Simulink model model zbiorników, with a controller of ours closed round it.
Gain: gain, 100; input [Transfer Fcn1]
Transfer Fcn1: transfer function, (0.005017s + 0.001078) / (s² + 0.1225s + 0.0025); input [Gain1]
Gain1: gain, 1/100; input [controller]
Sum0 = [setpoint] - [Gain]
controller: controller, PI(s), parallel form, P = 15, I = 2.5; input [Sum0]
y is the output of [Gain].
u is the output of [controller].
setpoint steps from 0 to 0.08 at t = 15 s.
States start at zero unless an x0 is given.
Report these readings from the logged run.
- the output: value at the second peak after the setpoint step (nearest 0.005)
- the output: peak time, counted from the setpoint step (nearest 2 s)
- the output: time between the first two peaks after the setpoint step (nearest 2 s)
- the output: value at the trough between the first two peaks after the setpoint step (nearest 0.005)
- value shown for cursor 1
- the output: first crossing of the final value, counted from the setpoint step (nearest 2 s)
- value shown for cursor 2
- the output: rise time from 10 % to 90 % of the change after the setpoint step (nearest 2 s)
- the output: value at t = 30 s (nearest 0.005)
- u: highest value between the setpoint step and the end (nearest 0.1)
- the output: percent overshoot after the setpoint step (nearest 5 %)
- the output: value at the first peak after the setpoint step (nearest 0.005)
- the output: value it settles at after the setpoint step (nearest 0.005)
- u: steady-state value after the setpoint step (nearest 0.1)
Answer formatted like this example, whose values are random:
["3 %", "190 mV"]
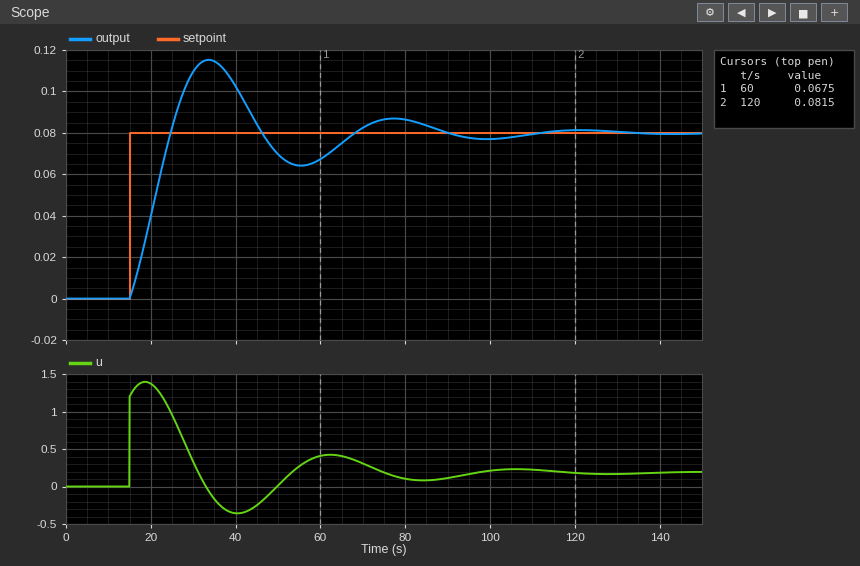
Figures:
["0.085", "18 s", "44 s", "0.065", "0.0675", "10 s", "0.0815", "8 s", "0.110", "1.4", "45 %", "0.115", "0.080", "0.2"]
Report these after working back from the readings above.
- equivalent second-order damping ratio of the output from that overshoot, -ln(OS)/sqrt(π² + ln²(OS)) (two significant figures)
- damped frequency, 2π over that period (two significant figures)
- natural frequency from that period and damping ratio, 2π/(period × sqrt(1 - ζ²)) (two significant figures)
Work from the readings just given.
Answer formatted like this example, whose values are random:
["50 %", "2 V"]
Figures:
["0.25", "0.14 rad/s", "0.15 rad/s"]
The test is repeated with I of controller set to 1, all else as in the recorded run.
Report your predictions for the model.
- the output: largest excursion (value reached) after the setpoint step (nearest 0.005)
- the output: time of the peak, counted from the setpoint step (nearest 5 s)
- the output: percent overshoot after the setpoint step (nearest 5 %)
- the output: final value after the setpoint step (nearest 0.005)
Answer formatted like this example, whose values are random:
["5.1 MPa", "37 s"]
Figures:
["0.100", "25 s", "25 %", "0.080"]
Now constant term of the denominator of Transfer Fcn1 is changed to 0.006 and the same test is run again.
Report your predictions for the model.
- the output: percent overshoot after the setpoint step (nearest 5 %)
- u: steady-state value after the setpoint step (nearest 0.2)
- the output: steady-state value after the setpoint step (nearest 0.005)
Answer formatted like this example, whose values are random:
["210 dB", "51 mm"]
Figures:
["35 %", "0.4", "0.080"]
